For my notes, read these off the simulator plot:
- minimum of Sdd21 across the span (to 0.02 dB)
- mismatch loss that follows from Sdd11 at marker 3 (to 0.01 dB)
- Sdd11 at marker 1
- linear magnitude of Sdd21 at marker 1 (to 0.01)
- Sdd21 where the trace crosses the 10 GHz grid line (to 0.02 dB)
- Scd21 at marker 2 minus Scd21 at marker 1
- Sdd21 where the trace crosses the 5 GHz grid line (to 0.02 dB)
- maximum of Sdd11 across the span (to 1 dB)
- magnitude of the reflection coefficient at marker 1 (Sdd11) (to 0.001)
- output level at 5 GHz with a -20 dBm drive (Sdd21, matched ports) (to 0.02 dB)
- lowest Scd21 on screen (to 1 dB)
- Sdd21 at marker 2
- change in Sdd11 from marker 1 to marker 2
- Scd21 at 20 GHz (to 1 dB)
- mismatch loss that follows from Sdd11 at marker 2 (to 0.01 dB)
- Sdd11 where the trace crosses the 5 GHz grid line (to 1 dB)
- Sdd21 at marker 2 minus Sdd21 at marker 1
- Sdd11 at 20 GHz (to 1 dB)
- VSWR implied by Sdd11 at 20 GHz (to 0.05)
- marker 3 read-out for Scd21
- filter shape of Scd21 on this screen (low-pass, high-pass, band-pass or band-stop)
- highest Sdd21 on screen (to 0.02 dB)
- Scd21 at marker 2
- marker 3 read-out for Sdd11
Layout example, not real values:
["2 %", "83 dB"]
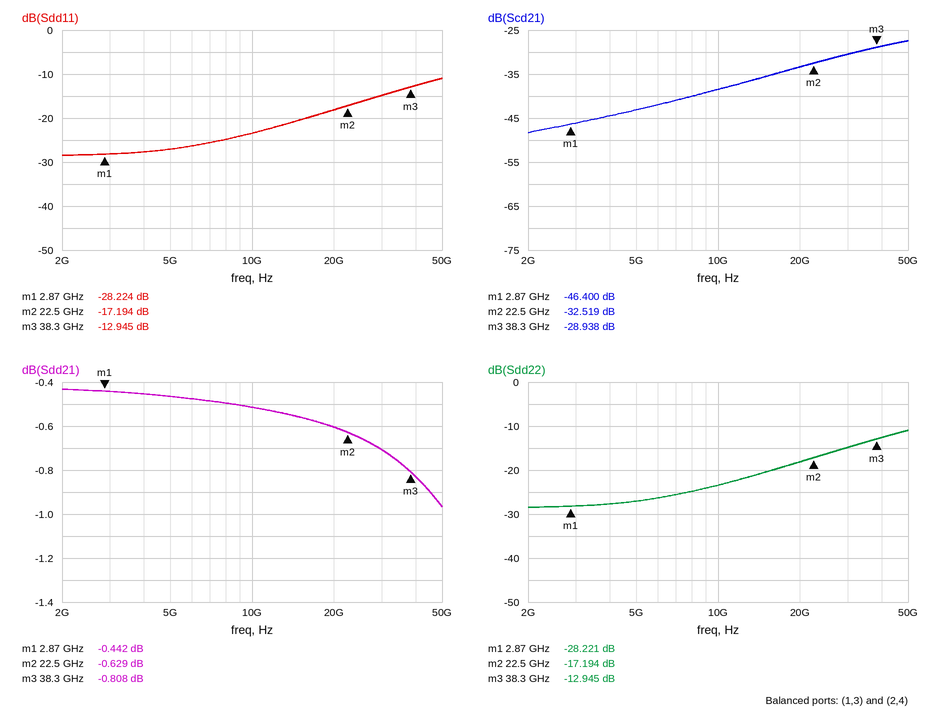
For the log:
["-0.96 dB", "0.23 dB", "-28.224 dB", "0.95", "-0.52 dB", "13.881 dB", "-0.46 dB", "-11 dB", "0.039", "-20.46 dBm", "-48 dB", "-0.629 dB", "11.030 dB", "-33 dB", "0.08 dB", "-27 dB", "-0.187 dB", "-18 dB", "1.30", "-28.938 dB", "high-pass", "-0.44 dB", "-32.519 dB", "-12.945 dB"]
